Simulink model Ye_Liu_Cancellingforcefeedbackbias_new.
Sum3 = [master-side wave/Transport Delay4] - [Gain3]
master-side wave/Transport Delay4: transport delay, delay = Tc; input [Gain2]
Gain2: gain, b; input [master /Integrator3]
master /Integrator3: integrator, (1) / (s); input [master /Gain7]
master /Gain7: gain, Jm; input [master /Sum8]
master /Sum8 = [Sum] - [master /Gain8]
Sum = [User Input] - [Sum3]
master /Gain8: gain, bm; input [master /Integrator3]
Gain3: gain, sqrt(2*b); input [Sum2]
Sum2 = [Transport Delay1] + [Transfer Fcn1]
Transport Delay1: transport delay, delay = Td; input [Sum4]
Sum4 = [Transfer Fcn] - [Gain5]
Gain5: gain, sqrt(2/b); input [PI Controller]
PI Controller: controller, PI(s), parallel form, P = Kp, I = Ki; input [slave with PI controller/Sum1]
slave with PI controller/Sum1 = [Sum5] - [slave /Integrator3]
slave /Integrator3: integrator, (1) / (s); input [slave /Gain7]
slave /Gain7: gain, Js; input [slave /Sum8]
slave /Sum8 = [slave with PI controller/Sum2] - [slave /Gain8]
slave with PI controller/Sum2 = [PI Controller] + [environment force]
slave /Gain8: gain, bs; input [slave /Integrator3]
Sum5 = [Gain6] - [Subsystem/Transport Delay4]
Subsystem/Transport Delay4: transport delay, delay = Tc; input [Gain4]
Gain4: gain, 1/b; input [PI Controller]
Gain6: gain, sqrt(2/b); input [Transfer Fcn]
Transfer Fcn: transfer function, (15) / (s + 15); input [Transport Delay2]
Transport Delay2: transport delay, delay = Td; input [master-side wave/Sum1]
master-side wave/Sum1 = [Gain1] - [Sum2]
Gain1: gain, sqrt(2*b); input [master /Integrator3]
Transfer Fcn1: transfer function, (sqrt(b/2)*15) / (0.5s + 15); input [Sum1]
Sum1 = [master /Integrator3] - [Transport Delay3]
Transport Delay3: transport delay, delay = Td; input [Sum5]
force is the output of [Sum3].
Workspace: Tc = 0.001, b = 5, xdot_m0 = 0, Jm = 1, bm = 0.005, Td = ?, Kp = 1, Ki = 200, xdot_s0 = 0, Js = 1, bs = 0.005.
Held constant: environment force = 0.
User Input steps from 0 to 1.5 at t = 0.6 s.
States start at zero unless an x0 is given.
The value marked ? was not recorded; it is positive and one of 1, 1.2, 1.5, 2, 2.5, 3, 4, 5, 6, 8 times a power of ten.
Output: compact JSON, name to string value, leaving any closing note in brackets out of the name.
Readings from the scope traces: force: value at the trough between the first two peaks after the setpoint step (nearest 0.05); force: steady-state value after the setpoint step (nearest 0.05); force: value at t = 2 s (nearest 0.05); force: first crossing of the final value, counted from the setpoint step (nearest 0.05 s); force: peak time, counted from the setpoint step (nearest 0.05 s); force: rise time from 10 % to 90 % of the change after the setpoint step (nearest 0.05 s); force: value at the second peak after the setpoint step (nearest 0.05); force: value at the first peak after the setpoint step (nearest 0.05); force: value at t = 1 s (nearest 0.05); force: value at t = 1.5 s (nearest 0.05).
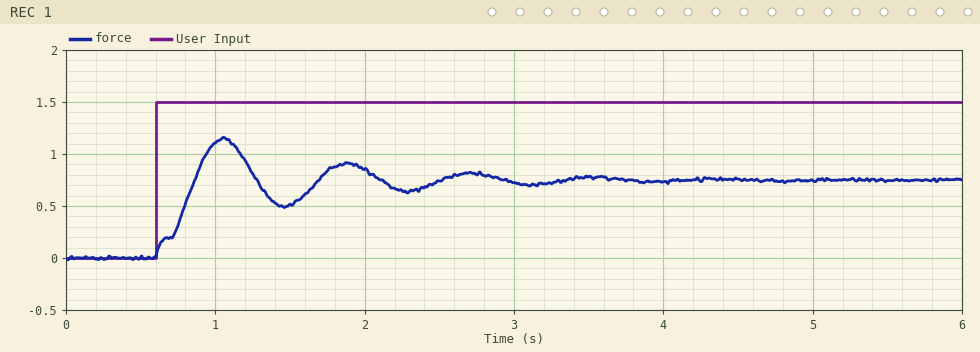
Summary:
{"force: value at the trough between the first two peaks after the setpoint step": "0.50", "force: steady-state value after the setpoint step": "0.75", "force: value at t = 2 s": "0.85", "force: first crossing of the final value, counted from the setpoint step": "0.25 s", "force: peak time, counted from the setpoint step": "0.45 s", "force: rise time from 10 % to 90 % of the change after the setpoint step": "0.25 s", "force: value at the second peak after the setpoint step": "0.90", "force: value at the first peak after the setpoint step": "1.15", "force: value at t = 1 s": "1.10", "force: value at t = 1.5 s": "0.50"}
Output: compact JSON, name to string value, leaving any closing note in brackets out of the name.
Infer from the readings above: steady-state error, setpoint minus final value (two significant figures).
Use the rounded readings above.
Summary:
{"steady-state error, setpoint minus final value": "0.75"}
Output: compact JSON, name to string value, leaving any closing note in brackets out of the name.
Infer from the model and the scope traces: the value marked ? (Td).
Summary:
{"the value marked ?": "0.04"}
